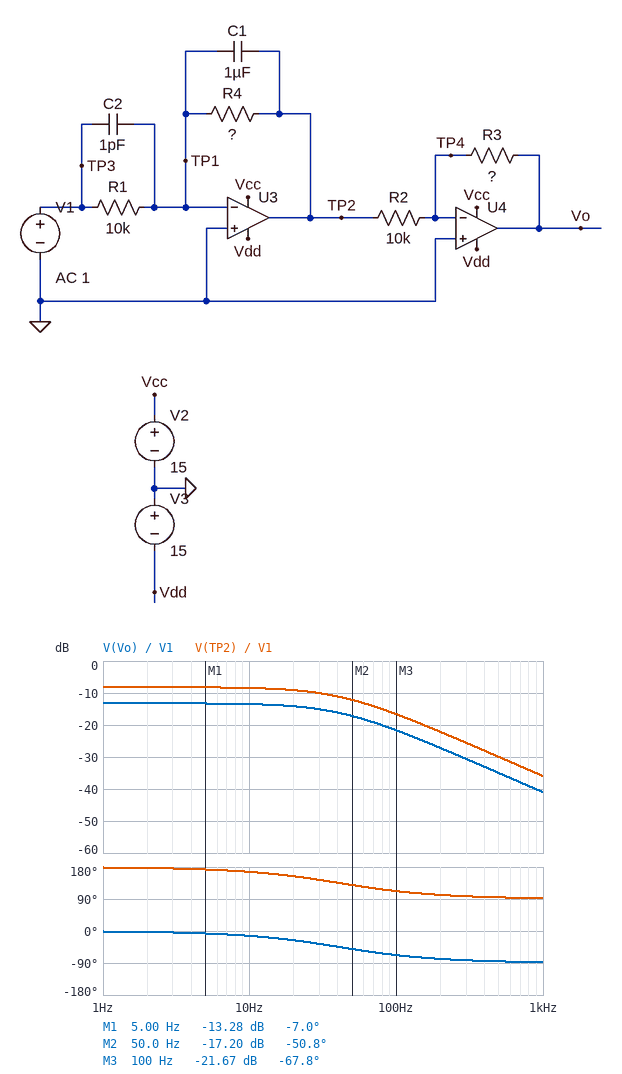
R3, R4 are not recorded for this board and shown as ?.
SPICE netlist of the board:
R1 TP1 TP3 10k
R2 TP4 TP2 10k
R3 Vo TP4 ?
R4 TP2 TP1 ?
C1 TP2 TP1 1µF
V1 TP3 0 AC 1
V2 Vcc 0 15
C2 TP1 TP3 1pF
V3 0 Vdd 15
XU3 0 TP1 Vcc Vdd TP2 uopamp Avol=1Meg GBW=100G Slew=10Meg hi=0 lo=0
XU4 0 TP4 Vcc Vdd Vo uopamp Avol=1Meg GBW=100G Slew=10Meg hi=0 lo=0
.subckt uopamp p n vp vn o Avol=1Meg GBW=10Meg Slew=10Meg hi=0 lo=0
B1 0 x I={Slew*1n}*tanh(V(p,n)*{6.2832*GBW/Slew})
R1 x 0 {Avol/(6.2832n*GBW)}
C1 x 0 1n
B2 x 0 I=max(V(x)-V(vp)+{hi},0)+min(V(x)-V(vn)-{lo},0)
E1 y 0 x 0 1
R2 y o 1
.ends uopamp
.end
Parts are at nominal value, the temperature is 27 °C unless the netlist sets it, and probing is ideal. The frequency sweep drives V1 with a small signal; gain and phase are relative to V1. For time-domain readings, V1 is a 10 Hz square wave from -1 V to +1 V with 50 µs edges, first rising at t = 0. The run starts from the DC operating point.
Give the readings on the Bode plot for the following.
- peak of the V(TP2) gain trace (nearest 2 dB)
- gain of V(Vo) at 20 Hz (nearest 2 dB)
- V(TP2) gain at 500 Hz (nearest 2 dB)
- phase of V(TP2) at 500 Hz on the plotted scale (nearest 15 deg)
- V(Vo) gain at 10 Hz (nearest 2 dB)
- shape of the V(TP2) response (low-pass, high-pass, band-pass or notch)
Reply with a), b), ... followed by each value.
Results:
a) -8 dB
b) -14 dB
c) -30 dB
d) 90 deg
e) -14 dB
f) low-pass
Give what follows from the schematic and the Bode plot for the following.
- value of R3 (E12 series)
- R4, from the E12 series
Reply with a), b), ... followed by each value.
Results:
a) 5.6 kΩ
b) 3.9 kΩ
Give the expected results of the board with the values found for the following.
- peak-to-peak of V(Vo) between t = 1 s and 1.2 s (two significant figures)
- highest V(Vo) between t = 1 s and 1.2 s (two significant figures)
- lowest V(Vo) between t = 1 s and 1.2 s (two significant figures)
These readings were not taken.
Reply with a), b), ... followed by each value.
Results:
a) 440 mV
b) 220 mV
c) -220 mV
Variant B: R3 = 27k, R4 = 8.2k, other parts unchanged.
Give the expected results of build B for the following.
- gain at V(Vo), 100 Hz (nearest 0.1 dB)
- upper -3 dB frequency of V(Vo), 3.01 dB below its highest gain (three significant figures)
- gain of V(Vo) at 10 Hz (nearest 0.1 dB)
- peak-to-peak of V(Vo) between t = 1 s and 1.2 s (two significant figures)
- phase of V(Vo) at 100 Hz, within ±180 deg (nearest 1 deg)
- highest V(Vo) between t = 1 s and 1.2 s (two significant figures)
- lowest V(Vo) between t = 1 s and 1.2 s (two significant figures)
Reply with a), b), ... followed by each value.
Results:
a) -7.5 dB
b) 19.4 Hz
c) 5.9 dB
d) 4.4 V
e) -79 deg
f) 2.2 V
g) -2.2 V
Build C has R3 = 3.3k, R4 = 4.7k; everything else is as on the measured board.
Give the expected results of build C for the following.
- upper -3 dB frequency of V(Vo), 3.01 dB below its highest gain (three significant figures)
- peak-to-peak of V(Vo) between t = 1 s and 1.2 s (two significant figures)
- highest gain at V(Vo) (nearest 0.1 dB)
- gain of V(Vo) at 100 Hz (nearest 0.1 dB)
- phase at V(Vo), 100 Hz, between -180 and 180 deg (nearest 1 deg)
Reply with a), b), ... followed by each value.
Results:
a) 33.9 Hz
b) 310 mV
c) -16.2 dB
d) -26.1 dB
e) -71 deg
